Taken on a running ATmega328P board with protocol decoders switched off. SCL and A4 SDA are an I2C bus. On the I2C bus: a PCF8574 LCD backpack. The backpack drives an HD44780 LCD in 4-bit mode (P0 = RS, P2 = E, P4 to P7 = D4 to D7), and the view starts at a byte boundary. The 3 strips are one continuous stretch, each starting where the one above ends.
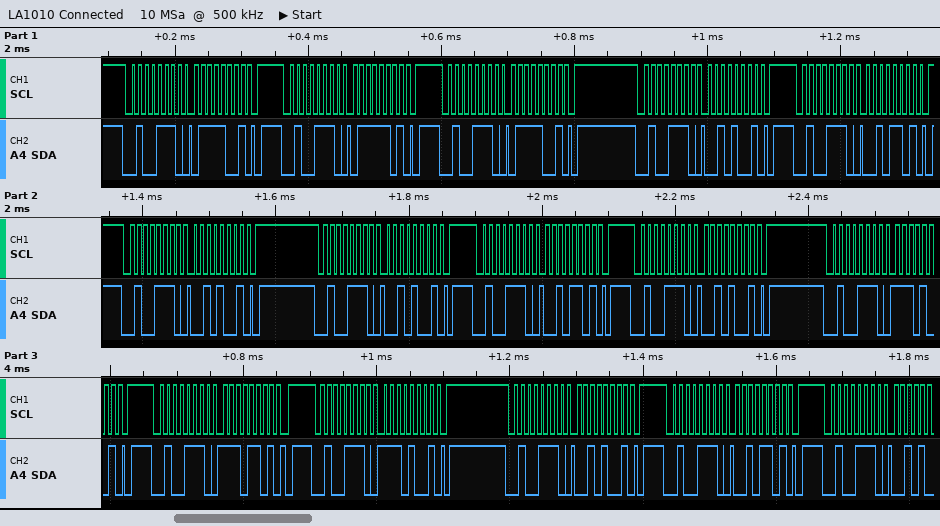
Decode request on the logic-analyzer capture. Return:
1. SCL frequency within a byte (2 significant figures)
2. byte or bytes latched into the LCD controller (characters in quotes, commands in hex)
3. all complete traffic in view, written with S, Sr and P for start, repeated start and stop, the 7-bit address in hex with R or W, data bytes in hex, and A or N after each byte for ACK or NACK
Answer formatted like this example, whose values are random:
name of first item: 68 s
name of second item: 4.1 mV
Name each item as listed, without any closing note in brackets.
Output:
SCL frequency within a byte: 100 kHz
byte or bytes latched into the LCD controller: 'r' '.'
all complete traffic in view, written with S, Sr and P for start, repeated start and stop, the 7-bit address in hex with R or W, data bytes in hex, and A or N after each byte for ACK or NACK: S 27W A 79 A P S 27W A 7D A P S 27W A 79 A P S 27W A 29 A P S 27W A 2D A P S 27W A 29 A P S 27W A 29 A P S 27W A 2D A P S 27W A 29 A P S 27W A E9 A P S 27W A ED A P S 27W A E9 A P S 27W A 29 A P S 27W A 2D A P S 27W A
